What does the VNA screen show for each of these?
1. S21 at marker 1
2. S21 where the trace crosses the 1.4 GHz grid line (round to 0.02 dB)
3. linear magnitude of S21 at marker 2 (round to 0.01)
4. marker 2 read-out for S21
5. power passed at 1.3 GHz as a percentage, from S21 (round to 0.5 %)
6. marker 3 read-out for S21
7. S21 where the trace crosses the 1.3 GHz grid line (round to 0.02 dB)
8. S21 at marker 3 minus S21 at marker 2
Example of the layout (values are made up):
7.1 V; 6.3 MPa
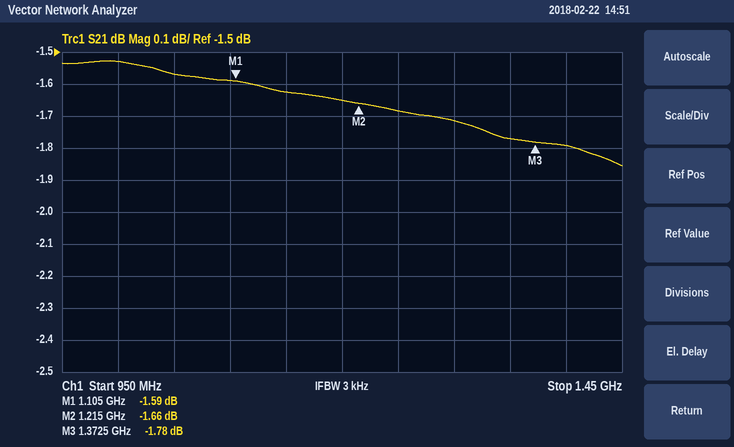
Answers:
-1.59 dB; -1.80 dB; 0.83; -1.66 dB; 67.5 %; -1.78 dB; -1.72 dB; -0.12 dB
